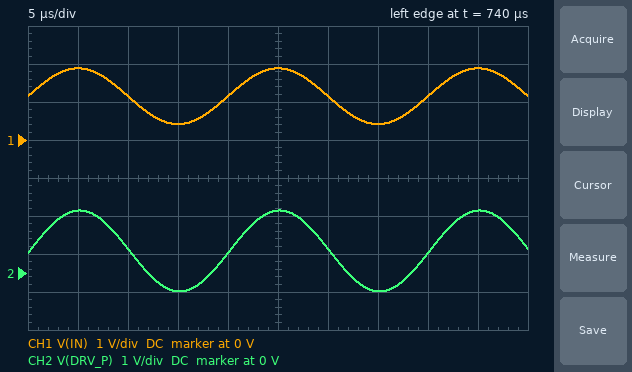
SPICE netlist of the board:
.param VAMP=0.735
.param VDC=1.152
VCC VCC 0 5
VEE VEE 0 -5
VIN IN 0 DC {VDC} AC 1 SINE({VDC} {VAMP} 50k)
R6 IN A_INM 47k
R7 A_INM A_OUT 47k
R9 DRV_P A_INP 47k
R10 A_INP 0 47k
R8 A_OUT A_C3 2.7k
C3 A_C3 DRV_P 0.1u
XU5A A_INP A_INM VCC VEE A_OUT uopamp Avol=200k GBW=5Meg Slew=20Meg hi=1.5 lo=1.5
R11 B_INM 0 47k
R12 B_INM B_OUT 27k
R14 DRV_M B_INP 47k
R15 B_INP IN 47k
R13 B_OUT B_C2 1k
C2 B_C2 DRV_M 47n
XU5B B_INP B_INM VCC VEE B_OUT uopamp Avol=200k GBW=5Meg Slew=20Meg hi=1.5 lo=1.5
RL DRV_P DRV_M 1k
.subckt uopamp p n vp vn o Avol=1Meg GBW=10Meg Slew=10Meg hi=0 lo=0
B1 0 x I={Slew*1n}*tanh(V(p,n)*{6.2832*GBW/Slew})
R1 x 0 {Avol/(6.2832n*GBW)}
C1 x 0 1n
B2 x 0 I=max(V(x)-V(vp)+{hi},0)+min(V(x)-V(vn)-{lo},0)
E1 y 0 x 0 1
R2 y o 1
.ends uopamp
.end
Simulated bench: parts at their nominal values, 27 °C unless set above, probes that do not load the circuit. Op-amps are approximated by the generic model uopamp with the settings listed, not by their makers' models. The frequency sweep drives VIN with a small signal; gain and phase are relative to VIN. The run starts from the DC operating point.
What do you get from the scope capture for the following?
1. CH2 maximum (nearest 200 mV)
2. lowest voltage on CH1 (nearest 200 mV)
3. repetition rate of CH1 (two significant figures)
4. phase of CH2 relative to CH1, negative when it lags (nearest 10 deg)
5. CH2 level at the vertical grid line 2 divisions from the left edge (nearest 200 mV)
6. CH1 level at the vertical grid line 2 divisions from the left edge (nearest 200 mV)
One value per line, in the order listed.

1.6 V
400 mV
50 kHz
0 deg
600 mV
1.2 V
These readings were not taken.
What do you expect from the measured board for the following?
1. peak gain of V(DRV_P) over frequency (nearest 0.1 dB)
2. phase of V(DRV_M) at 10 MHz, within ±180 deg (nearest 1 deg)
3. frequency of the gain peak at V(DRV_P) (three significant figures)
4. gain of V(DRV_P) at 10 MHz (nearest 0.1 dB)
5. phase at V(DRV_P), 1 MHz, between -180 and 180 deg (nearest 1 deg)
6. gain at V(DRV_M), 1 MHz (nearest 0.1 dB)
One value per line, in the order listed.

11.2 dB
-79 deg
442 Hz
-28.1 dB
-74 deg
-0.9 dB
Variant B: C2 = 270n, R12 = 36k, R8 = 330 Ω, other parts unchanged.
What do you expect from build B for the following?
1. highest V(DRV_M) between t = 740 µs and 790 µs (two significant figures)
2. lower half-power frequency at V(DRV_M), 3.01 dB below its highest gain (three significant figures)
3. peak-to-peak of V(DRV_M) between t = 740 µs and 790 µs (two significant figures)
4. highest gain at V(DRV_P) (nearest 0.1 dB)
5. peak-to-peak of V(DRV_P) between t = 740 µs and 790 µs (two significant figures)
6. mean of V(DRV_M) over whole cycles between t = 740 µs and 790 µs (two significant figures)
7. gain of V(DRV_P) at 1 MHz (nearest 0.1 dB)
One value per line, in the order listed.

3.4 V
4.21 kHz
5.2 V
25.0 dB
6.5 V
660 mV
3.9 dB
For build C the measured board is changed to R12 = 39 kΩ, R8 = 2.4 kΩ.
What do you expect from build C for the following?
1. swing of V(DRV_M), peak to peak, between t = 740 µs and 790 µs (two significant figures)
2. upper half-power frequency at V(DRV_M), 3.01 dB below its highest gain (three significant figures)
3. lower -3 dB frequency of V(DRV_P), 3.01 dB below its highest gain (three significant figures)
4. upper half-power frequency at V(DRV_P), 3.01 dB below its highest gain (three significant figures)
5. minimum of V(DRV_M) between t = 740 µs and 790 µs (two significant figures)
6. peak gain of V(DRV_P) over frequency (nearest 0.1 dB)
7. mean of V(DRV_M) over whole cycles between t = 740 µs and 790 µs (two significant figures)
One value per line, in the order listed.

4.7 V
120 kHz
308 Hz
67.4 kHz
-2.3 V
15.3 dB
540 mV
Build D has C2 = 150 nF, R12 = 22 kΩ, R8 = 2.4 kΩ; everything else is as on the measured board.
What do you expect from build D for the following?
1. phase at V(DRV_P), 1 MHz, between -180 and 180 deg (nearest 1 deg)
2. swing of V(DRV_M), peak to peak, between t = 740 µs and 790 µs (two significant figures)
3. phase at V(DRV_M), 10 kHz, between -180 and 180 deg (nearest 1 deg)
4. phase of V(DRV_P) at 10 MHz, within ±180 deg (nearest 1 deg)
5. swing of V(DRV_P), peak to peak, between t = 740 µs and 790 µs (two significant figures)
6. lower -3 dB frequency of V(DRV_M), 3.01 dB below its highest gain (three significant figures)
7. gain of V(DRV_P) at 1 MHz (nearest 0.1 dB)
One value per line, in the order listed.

-69 deg
1.7 V
2 deg
-83 deg
1.1 V
674 Hz
-9.3 dB
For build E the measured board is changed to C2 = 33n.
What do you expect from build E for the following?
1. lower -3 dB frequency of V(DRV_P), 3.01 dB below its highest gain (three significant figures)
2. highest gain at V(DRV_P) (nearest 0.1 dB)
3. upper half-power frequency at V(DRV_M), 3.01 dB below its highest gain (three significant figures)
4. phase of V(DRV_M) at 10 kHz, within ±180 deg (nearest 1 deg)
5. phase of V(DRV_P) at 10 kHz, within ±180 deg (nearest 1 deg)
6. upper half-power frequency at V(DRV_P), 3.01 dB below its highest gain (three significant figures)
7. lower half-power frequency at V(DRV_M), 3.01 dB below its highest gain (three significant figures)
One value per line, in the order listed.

209 Hz
14.5 dB
1.39 kHz
21 deg
25 deg
1.32 kHz
211 Hz
